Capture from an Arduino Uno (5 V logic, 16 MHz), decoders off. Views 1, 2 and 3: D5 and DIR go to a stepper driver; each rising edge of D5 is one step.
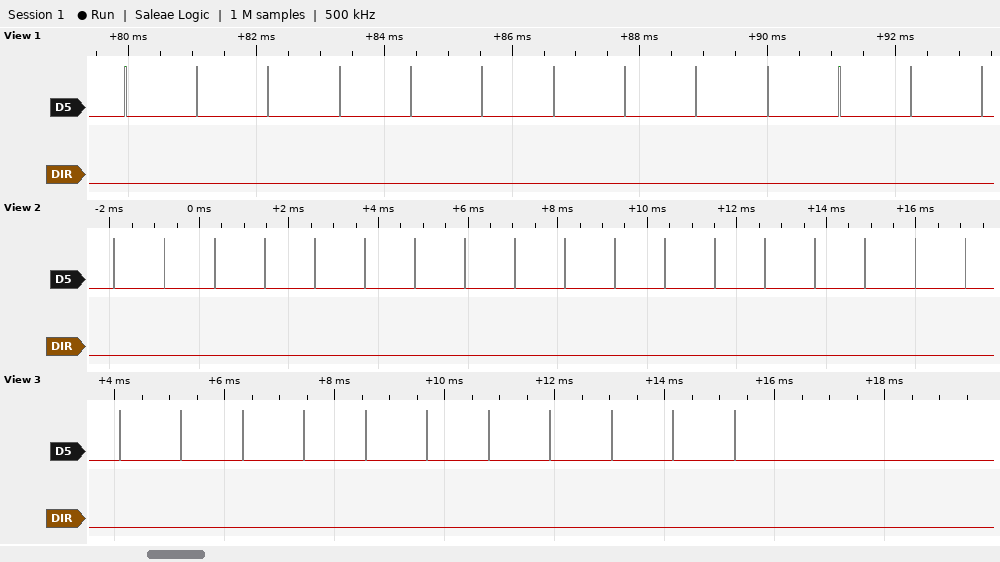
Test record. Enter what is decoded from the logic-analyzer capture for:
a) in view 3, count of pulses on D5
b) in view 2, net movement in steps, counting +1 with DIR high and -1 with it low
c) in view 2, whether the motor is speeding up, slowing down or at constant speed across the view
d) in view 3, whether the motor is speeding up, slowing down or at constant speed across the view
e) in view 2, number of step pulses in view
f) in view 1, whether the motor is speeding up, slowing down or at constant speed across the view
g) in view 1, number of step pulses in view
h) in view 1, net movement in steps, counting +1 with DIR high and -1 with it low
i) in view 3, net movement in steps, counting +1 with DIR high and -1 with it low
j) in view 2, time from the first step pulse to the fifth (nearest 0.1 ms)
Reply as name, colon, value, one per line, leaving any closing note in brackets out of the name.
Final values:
in view 3, count of pulses on D5: 11
in view 2, net movement in steps, counting +1 with DIR high and -1 with it low: -18
in view 2, whether the motor is speeding up, slowing down or at constant speed across the view: constant speed
in view 3, whether the motor is speeding up, slowing down or at constant speed across the view: constant speed
in view 2, number of step pulses in view: 18
in view 1, whether the motor is speeding up, slowing down or at constant speed across the view: constant speed
in view 1, number of step pulses in view: 13
in view 1, net movement in steps, counting +1 with DIR high and -1 with it low: -13
in view 3, net movement in steps, counting +1 with DIR high and -1 with it low: -11
in view 2, time from the first step pulse to the fifth: 4.5 ms
